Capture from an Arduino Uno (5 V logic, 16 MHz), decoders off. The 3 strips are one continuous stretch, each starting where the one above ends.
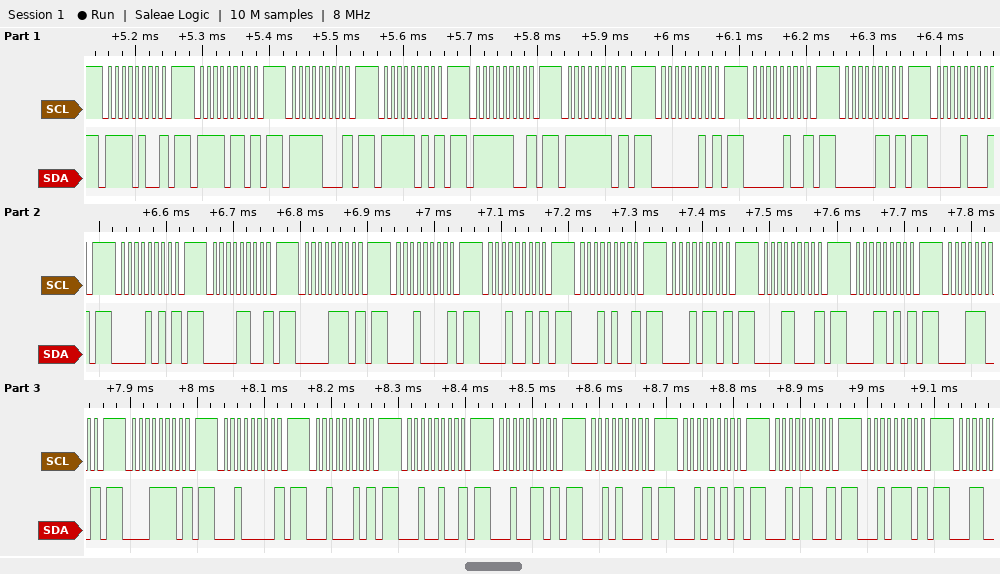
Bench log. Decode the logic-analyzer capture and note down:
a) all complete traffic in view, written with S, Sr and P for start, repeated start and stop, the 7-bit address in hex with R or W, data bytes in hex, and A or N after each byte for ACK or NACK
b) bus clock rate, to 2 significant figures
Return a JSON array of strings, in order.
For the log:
["S 7AW N P S 7BW N P S 7CW N P S 7DW N P S 7EW N P S 7FW N P S 01W N P S 02W N P S 03W N P S 04W N P S 05W N P S 06W N P S 07W N P S 08W N P S 09W N P S 0AW N P S 0BW N P S 0CW N P S 0DW N P S 0EW N P S 0FW N P S 10W N P S 11W N P S 12W N P S 13W N P S 14W N P S 15W N P S 16W N P S 17W N P", "100 kHz"]
